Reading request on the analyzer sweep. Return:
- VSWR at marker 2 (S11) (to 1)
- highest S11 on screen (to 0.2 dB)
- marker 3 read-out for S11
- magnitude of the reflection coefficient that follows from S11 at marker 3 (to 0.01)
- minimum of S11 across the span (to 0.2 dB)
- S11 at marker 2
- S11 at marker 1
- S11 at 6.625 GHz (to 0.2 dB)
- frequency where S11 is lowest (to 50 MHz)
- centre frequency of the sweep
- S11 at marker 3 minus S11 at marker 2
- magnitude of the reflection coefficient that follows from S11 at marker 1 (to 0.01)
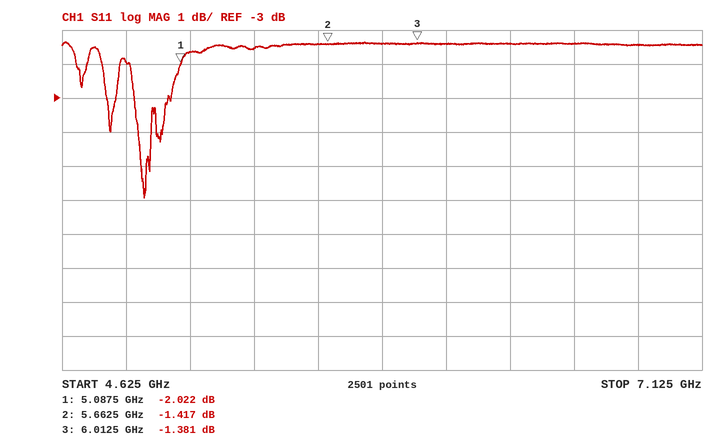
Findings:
12
-1.4 dB
-1.381 dB
0.85
-6.0 dB
-1.417 dB
-2.022 dB
-1.4 dB
4.95 GHz
5.875 GHz
0.036 dB
0.79
